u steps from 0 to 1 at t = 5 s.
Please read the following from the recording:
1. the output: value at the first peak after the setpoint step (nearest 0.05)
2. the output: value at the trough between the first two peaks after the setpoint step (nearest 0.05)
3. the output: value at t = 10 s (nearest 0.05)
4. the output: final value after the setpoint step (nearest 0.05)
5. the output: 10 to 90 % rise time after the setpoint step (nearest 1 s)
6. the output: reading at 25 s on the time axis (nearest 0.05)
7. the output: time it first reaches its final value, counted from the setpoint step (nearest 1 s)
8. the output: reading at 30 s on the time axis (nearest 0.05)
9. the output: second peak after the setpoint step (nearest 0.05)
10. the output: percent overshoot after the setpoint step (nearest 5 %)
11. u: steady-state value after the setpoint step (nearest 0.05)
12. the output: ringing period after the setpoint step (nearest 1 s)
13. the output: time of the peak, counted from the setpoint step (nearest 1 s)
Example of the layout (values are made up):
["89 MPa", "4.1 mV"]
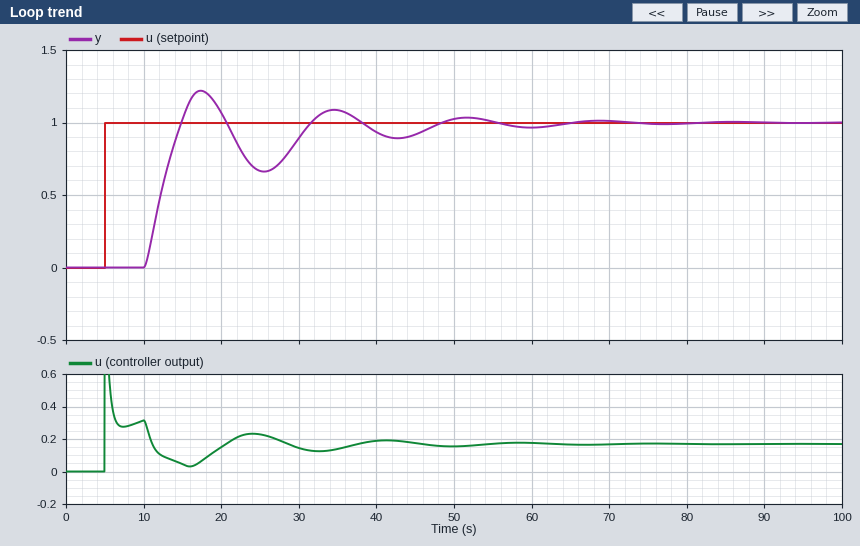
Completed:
["1.20", "0.65", "0.00", "1.00", "4 s", "0.65", "10 s", "0.90", "1.10", "20 %", "0.15", "17 s", "12 s"]
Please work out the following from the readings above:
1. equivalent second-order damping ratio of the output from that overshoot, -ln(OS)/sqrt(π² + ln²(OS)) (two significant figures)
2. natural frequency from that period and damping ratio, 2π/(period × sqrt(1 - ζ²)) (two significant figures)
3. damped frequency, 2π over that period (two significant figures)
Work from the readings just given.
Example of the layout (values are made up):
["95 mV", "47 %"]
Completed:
["0.46", "0.42 rad/s", "0.37 rad/s"]
